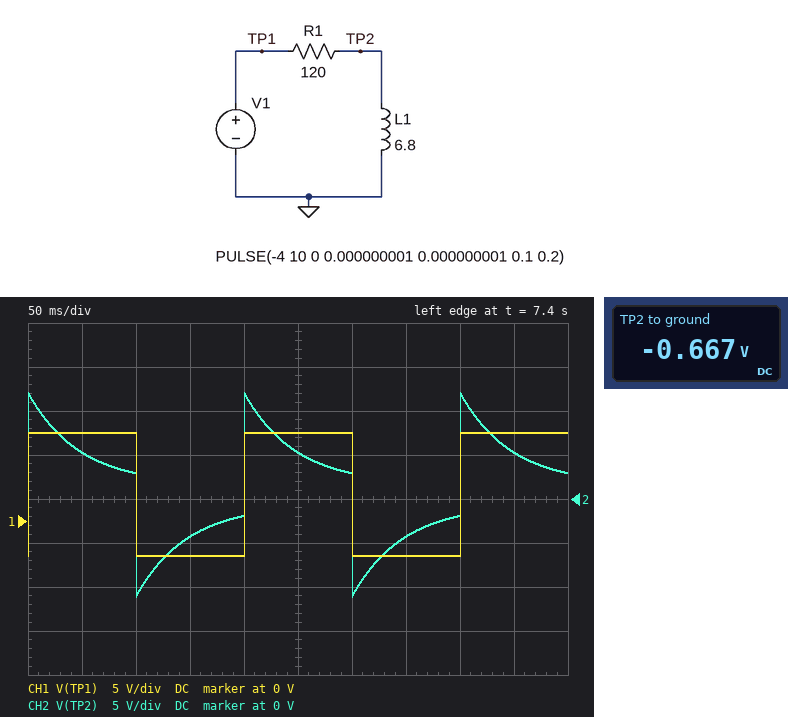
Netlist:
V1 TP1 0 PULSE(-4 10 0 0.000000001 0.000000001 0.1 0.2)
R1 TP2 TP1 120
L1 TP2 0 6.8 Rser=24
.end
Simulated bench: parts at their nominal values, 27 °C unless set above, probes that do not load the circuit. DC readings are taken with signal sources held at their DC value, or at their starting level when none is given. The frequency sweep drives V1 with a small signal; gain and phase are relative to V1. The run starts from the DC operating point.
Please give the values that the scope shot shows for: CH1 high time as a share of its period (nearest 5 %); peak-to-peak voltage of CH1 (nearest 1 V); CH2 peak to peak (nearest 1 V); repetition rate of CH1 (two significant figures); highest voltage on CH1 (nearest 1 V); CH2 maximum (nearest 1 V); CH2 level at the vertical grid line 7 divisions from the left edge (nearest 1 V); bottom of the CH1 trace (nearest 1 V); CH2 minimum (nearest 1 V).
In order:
50 %
14 V
23 V
5.0 Hz
10 V
12 V
-4 V
-4 V
-11 V
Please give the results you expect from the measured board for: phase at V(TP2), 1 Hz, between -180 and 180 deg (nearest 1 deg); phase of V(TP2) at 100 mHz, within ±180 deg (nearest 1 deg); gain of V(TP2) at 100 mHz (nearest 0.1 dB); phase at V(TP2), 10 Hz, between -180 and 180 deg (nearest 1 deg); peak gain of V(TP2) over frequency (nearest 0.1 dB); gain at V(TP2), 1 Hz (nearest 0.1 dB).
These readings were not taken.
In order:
44 deg
8 deg
-15.4 dB
15 deg
0 dB
-9.7 dB
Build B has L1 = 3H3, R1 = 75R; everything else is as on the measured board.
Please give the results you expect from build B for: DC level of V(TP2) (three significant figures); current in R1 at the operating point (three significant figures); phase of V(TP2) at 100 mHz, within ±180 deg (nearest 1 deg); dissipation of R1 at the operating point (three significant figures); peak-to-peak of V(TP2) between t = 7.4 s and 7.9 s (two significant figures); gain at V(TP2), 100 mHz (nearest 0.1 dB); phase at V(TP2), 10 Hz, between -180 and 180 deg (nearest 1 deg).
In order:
-970 mV
40.4 mA
4 deg
122 mW
24 V
-12.3 dB
19 deg
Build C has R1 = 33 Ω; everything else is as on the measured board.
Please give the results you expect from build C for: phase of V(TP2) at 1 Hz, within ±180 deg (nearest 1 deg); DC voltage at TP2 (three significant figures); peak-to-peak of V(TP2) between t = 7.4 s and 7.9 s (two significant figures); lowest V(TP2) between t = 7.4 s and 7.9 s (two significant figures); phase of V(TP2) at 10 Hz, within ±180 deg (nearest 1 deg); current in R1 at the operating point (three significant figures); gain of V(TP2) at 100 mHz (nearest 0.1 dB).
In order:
24 deg
-1.68 V
17 V
-7.3 V
4 deg
70.2 mA
-7.4 dB
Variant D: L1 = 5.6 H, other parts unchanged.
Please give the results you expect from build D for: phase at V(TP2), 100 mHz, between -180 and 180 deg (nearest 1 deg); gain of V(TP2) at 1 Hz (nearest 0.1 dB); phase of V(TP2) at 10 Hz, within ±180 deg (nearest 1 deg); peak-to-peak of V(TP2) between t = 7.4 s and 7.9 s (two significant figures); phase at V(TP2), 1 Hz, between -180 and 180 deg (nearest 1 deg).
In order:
7 deg
-10.8 dB
18 deg
24 V
42 deg
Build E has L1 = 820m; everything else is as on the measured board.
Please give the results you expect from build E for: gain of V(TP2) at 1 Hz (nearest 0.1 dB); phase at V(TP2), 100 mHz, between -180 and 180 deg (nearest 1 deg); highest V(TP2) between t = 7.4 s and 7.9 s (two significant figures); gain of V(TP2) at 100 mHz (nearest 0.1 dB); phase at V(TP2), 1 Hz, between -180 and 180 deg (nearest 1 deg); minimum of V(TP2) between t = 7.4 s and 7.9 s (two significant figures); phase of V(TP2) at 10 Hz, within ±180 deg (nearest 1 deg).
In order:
-15.4 dB
1 deg
13 V
-15.6 dB
10 deg
-12 V
45 deg
